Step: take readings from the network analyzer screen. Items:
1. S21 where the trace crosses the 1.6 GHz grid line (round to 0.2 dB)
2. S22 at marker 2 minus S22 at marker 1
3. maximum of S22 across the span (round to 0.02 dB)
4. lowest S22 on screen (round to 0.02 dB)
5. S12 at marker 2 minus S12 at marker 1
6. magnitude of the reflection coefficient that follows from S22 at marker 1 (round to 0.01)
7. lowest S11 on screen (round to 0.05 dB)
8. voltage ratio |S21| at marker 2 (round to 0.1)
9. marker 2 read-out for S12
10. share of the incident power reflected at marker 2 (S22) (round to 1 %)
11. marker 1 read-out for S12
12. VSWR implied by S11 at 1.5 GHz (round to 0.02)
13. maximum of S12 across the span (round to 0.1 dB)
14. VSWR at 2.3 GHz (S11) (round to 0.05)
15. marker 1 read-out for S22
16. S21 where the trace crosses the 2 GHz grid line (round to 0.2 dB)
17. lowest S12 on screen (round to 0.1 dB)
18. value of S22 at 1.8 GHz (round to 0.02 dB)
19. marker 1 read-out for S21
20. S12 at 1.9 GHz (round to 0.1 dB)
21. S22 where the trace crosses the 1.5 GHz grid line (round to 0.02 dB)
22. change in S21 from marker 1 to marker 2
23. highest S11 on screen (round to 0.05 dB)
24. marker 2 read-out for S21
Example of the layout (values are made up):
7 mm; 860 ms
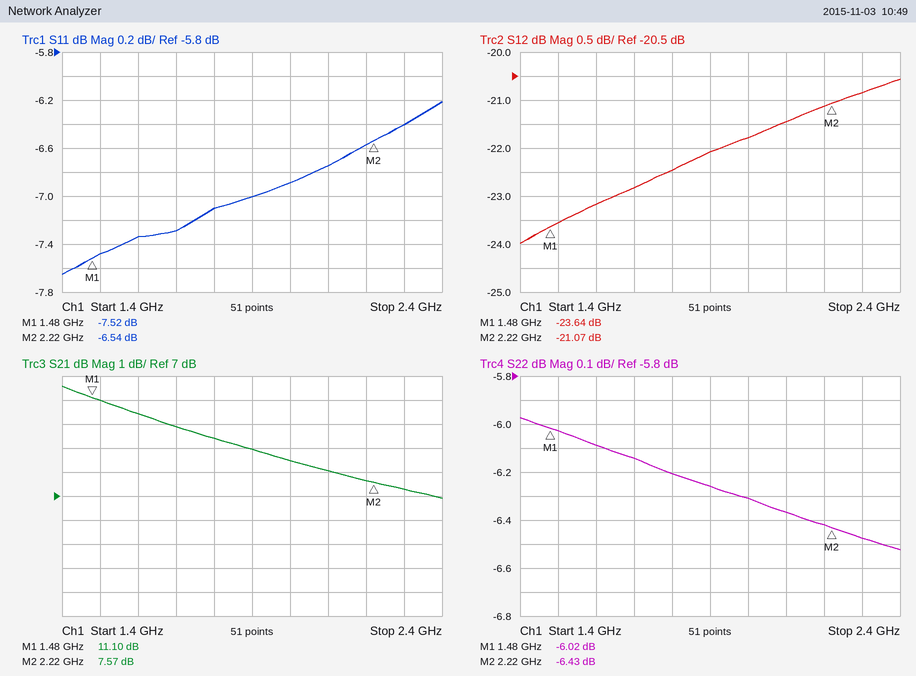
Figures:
10.4 dB; -0.41 dB; -5.98 dB; -6.52 dB; 2.57 dB; 0.50; -7.65 dB; 2.4; -21.07 dB; 23 %; -23.64 dB; 2.46; -20.6 dB; 2.85; -6.02 dB; 8.4 dB; -24.0 dB; -6.20 dB; 11.10 dB; -22.1 dB; -6.02 dB; -3.53 dB; -6.20 dB; 7.57 dB
